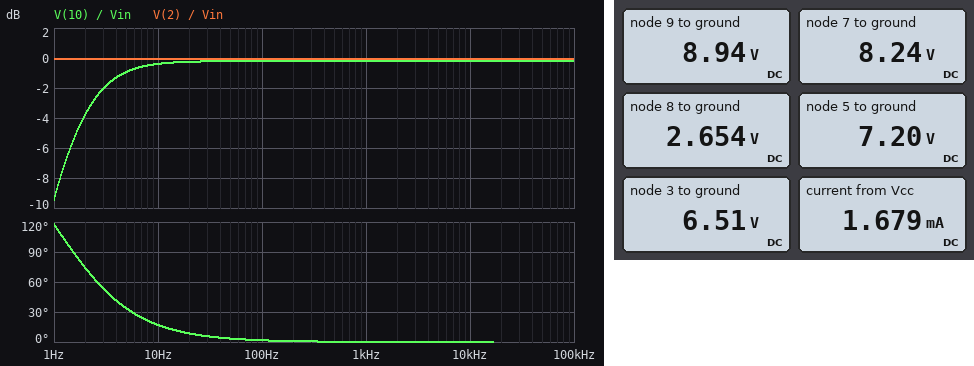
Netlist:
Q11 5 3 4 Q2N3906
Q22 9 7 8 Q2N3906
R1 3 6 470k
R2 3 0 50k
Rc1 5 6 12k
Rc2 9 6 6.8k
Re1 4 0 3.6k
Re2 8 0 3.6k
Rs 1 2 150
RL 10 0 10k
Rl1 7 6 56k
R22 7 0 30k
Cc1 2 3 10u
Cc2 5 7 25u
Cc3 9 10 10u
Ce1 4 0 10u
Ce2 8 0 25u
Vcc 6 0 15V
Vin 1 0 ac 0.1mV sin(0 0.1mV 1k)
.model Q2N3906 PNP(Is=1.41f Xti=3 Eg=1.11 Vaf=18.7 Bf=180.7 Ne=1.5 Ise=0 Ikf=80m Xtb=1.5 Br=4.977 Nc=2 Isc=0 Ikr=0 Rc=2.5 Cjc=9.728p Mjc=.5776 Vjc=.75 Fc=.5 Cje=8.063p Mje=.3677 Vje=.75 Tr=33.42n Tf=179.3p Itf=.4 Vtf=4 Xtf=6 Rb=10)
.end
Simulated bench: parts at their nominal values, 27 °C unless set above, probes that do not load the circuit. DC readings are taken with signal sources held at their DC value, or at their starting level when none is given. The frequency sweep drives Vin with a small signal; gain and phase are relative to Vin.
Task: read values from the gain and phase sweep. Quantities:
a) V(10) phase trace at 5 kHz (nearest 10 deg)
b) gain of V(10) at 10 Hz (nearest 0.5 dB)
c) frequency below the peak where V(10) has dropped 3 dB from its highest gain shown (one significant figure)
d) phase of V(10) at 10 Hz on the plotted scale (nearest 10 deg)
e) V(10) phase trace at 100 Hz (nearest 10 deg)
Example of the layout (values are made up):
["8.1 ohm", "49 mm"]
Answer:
["0 deg", "-0.5 dB", "2 Hz", "20 deg", "0 deg"]
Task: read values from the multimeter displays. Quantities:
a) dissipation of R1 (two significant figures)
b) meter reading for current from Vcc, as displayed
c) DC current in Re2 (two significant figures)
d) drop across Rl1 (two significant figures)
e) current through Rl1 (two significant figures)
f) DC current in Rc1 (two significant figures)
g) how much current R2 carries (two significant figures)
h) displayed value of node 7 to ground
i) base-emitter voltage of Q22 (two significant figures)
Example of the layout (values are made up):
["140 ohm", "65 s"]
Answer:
["150 µW", "1.679 mA", "740 µA", "6.8 V", "120 µA", "650 µA", "130 µA", "8.24 V", "5.6 V"]
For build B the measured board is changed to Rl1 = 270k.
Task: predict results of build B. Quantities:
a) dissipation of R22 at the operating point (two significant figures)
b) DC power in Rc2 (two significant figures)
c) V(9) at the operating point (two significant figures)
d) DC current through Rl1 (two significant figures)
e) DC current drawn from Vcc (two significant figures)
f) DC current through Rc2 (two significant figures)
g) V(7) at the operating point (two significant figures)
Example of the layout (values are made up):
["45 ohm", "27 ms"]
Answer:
["1.5 mW", "8.5 mW", "7.4 V", "31 µA", "1.8 mA", "1.1 mA", "6.7 V"]
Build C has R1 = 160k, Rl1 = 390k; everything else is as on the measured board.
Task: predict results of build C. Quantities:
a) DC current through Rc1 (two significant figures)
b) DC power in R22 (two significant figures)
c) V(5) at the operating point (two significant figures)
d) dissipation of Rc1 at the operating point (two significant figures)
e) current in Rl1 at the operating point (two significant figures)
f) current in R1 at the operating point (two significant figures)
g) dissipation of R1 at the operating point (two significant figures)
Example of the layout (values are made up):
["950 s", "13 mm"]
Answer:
["580 µA", "1.4 mW", "8.1 V", "4.0 mW", "22 µA", "48 µA", "360 µW"]
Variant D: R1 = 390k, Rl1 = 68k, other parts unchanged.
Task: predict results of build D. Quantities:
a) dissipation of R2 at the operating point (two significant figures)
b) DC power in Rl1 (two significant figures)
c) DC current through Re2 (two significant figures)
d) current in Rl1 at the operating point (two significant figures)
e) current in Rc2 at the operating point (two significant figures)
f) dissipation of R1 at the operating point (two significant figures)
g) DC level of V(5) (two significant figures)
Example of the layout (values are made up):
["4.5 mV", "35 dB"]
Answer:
["870 µW", "730 µW", "770 µA", "100 µA", "930 µA", "180 µW", "7.3 V"]
